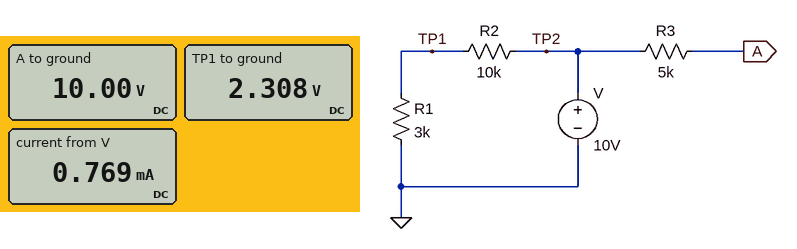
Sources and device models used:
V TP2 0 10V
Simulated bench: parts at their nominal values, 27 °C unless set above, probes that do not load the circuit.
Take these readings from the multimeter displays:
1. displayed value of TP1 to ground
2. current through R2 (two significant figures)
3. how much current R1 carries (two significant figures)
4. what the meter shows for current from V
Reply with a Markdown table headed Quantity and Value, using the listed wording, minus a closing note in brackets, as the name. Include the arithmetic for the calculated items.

| Quantity | Value |
|---|---|
| displayed value of TP1 to ground | 2.308 V |
| current through R2 | (10 V - 2.308 V) / 10 kΩ = 770 µA |
| how much current R1 carries | (2.308 V) / 3 kΩ = 770 µA |
| what the meter shows for current from V | 0.769 mA |
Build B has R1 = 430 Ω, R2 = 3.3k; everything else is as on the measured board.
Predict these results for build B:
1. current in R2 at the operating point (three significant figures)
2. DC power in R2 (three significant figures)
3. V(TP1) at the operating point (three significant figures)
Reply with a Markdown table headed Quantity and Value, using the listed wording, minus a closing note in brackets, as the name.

| Quantity | Value |
|---|---|
| current in R2 at the operating point | 2.68 mA |
| DC power in R2 | 23.7 mW |
| V(TP1) at the operating point | 1.15 V |
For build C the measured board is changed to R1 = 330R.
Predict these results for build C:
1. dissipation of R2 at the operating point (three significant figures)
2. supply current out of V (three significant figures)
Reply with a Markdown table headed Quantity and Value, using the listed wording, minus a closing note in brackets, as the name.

| Quantity | Value |
|---|---|
| dissipation of R2 at the operating point | 9.37 mW |
| supply current out of V | 968 µA |
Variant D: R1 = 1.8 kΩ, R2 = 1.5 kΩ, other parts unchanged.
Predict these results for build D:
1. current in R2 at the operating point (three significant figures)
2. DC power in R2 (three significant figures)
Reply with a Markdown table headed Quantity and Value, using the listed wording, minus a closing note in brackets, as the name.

| Quantity | Value |
|---|---|
| current in R2 at the operating point | 3.03 mA |
| DC power in R2 | 13.8 mW |
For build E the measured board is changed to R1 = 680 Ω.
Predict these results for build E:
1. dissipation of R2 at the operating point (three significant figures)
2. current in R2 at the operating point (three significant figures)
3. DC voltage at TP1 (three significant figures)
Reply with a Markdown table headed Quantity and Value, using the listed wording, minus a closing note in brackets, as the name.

| Quantity | Value |
|---|---|
| dissipation of R2 at the operating point | 8.77 mW |
| current in R2 at the operating point | 936 µA |
| DC voltage at TP1 | 637 mV |
